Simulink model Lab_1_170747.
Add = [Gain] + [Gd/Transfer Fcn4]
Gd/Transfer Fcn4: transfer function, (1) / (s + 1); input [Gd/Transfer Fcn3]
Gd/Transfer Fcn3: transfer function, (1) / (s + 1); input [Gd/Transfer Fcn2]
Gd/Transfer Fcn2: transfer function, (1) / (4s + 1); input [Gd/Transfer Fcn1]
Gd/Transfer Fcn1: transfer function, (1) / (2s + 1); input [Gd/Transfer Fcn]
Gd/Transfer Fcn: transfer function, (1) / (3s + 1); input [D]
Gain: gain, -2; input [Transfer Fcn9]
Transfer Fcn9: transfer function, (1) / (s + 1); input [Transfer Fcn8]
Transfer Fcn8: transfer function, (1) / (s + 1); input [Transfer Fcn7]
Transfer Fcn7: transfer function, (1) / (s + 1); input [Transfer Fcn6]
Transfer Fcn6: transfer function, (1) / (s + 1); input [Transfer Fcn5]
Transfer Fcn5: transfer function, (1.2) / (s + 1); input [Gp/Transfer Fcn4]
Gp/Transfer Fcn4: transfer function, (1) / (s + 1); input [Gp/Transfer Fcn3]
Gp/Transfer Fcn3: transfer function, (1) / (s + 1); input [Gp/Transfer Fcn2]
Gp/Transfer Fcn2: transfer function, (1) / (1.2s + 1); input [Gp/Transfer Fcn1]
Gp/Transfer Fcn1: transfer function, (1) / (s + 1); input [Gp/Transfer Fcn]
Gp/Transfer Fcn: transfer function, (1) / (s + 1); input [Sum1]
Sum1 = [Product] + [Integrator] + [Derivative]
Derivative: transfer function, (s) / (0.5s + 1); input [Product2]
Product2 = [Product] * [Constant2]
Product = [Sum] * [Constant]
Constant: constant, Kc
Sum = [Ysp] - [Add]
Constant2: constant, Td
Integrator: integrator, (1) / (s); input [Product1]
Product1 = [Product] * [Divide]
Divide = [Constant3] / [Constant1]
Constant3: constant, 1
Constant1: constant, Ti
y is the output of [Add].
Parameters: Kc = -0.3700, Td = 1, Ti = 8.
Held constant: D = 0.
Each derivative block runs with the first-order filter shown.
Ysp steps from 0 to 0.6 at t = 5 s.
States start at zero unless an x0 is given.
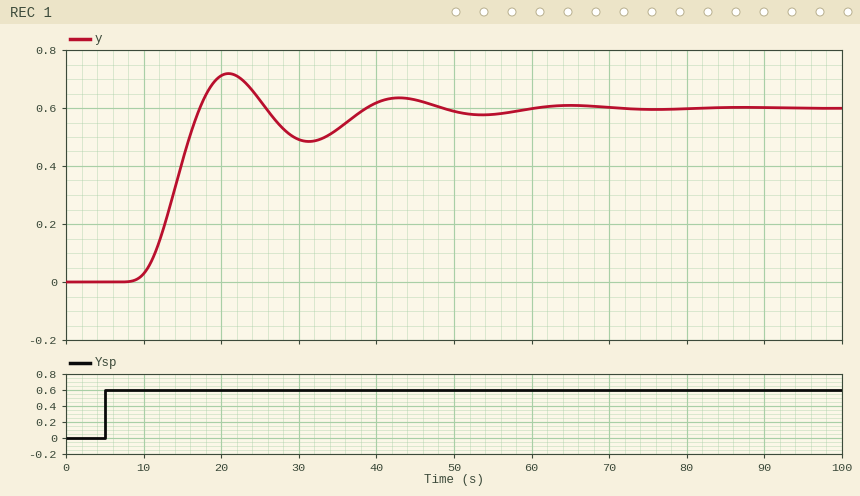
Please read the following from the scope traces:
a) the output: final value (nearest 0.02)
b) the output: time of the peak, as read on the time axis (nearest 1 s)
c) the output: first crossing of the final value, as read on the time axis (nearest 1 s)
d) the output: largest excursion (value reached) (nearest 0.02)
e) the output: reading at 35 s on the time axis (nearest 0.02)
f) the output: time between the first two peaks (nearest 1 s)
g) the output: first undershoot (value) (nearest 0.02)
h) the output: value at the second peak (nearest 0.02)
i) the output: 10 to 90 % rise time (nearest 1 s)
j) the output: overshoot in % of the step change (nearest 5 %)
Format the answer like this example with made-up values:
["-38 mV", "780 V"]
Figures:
["0.60", "21 s", "17 s", "0.72", "0.52", "22 s", "0.48", "0.64", "6 s", "20 %"]
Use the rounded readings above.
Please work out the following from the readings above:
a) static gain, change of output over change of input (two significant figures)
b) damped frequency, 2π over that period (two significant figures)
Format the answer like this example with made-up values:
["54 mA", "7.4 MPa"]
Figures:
["1.0", "0.29 rad/s"]
